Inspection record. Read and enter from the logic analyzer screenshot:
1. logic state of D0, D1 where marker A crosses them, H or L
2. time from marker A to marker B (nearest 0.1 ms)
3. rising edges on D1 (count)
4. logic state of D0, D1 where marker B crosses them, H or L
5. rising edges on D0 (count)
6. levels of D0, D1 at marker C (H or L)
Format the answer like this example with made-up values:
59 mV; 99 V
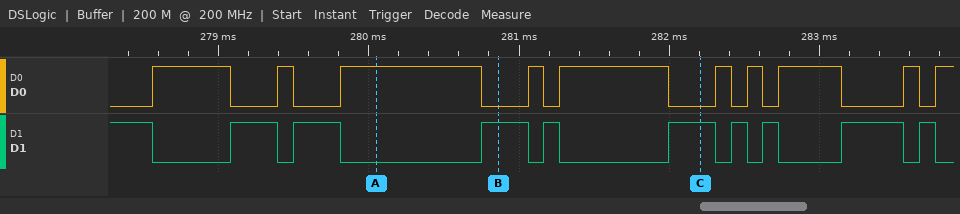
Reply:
D0=H, D1=L; 0.8 ms; 9; D0=L, D1=H; 10; D0=L, D1=H
